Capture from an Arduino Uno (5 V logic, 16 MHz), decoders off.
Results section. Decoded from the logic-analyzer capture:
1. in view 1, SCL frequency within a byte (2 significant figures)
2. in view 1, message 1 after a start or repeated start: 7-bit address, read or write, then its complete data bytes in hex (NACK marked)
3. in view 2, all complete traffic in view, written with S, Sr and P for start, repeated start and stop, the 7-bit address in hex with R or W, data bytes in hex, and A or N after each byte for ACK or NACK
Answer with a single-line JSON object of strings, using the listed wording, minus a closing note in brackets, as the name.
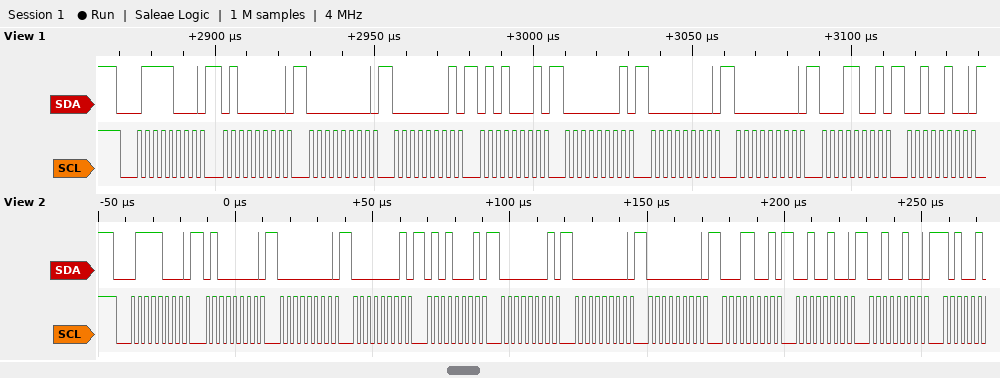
{"in view 1, SCL frequency within a byte": "400 kHz", "in view 1, message 1 after a start or repeated start: 7-bit address, read or write, then its complete data bytes in hex": "0x3C write: 40 00 01 51 01 00 00 19 24", "in view 2, all complete traffic in view, written with S, Sr and P for start, repeated start and stop, the 7-bit address in hex with R or W, data bytes in hex, and A or N after each byte for ACK or NACK": "S 3CW A 40 A 00 A 01 A 51 A 01 A 00 A 00 A 19 A 24 A 24 A"}
